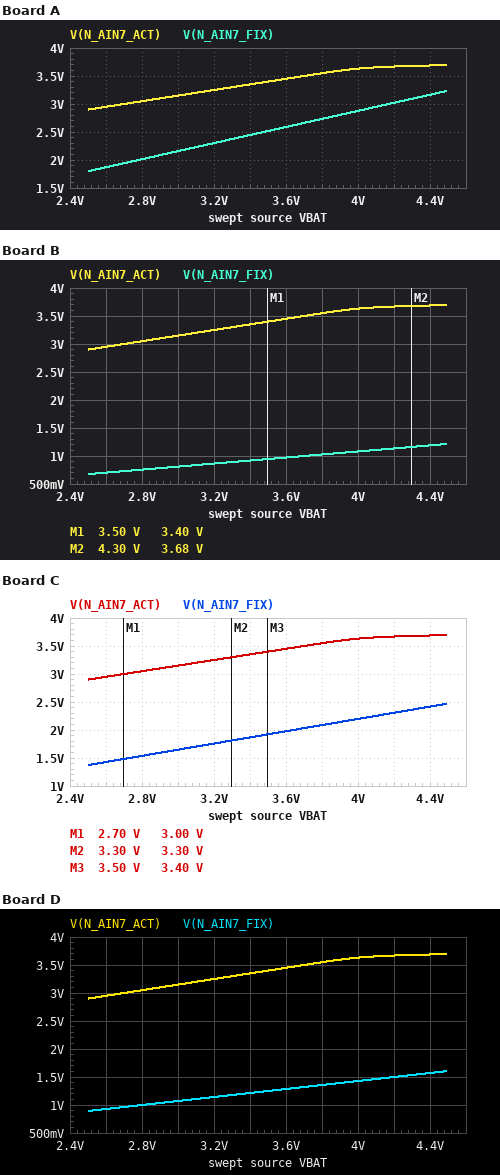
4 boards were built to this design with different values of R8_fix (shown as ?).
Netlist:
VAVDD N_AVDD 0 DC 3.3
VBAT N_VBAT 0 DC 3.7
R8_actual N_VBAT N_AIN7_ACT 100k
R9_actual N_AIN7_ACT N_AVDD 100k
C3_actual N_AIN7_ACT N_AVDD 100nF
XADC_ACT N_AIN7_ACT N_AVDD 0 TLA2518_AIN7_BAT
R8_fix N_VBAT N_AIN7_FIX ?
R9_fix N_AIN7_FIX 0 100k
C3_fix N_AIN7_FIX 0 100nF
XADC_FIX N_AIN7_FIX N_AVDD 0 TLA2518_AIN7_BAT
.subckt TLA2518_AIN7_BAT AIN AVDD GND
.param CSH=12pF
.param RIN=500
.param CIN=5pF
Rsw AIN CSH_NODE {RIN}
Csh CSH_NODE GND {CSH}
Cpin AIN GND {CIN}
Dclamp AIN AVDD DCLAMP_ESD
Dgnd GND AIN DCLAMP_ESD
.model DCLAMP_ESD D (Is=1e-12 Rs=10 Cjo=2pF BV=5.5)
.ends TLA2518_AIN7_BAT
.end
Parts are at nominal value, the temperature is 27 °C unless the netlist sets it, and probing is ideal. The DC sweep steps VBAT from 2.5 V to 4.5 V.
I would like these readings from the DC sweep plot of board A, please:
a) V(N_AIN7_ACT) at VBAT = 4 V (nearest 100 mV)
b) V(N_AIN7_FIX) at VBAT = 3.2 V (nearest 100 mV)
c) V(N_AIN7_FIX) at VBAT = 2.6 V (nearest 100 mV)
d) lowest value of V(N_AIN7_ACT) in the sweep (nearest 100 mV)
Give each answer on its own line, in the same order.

3.6 V
2.3 V
1.9 V
2.9 V
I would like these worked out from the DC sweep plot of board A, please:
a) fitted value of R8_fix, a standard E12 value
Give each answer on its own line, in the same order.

39 kΩ
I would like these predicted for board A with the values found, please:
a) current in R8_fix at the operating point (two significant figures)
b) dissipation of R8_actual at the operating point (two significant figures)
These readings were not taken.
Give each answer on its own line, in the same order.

27 µA
400 nW
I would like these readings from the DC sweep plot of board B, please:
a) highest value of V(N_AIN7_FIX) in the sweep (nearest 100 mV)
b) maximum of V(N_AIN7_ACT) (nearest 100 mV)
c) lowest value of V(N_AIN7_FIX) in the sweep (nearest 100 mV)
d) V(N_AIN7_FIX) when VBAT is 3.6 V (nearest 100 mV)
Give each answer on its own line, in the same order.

1.2 V
3.7 V
700 mV
1.0 V
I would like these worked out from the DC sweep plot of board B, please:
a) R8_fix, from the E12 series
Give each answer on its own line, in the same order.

270 kΩ
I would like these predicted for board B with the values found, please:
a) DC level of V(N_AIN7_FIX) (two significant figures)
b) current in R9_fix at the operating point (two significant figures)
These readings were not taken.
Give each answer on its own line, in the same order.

1.0 V
10 µA
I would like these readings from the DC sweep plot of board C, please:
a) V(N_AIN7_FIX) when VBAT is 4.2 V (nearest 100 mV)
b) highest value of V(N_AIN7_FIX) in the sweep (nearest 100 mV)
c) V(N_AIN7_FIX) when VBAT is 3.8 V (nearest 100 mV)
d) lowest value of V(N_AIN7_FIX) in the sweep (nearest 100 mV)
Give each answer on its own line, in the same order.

2.3 V
2.5 V
2.1 V
1.4 V
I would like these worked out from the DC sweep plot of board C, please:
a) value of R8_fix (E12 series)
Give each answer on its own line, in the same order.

82 kΩ
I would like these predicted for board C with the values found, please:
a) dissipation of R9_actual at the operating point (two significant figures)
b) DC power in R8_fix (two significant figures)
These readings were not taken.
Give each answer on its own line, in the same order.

400 nW
34 µW
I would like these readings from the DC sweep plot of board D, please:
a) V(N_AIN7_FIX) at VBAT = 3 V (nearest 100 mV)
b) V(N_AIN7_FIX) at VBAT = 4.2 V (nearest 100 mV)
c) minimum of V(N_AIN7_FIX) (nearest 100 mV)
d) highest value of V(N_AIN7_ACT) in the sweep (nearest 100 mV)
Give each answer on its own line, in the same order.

1.1 V
1.5 V
900 mV
3.7 V
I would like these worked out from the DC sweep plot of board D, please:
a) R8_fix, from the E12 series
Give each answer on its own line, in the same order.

180 kΩ
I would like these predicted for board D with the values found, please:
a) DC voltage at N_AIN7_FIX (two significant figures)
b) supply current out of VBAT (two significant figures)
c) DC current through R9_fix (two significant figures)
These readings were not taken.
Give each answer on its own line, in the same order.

1.3 V
15 µA
13 µA
